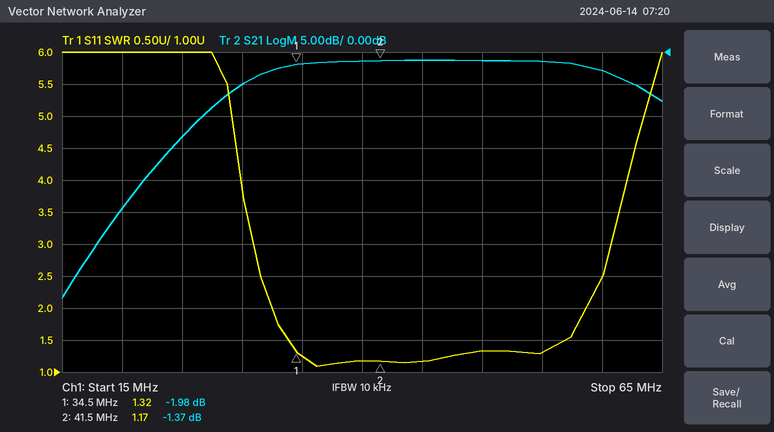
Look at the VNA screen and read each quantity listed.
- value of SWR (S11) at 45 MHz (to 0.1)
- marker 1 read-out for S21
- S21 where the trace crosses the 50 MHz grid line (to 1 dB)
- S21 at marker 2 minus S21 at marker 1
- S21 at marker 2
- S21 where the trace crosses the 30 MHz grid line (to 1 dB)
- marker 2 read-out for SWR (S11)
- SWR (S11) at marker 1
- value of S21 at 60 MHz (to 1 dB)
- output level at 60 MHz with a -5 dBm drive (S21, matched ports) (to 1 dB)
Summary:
1.2
-1.98 dB
-1 dB
0.61 dB
-1.37 dB
-5 dB
1.17
1.32
-3 dB
-8 dBm
